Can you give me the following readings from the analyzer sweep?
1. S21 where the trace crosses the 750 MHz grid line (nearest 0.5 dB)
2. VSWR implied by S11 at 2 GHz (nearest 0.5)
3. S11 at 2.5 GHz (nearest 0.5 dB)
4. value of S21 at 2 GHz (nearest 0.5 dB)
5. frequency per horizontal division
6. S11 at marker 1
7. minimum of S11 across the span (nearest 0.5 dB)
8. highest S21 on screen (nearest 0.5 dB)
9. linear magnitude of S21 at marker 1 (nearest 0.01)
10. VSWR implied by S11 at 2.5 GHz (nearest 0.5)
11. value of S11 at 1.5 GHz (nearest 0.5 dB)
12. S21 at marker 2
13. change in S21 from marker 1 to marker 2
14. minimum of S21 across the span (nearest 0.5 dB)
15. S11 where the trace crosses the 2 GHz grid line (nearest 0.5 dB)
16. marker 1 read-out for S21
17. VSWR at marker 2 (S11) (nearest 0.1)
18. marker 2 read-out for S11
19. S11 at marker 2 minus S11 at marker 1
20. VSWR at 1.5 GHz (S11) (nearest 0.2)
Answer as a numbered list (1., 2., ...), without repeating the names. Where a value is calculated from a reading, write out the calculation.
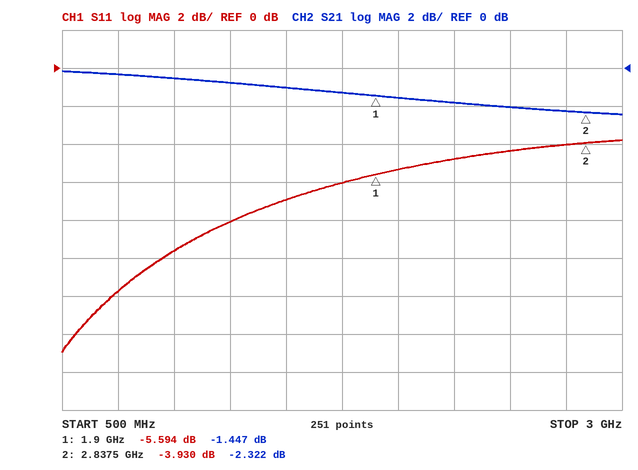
1. -0.5 dB
2. |Γ| = 10^(-5.5/20) = 0.5309; VSWR = (1 + 0.5309)/(1 − 0.5309) ≈ 3.26, so 3.5 to the nearest 0.5
3. -4.5 dB
4. -1.5 dB
5. 250 MHz
6. -5.594 dB
7. -15.0 dB
8. 0.0 dB
9. 10^(-1.447/20) ≈ 0.85
10. |Γ| = 10^(-4.5/20) = 0.5957; VSWR = (1 + 0.5957)/(1 − 0.5957) ≈ 4.0
11. -7.0 dB
12. -2.322 dB
13. -2.322 − (-1.447) = -0.875 dB
14. -2.5 dB
15. -5.5 dB
16. -1.447 dB
17. (1 + 0.6361)/(1 − 0.6361) ≈ 4.5
18. -3.930 dB
19. -3.93 − (-5.594) = 1.664 dB
20. |Γ| = 10^(-7/20) = 0.4467; VSWR = (1 + 0.4467)/(1 − 0.4467) ≈ 2.6
